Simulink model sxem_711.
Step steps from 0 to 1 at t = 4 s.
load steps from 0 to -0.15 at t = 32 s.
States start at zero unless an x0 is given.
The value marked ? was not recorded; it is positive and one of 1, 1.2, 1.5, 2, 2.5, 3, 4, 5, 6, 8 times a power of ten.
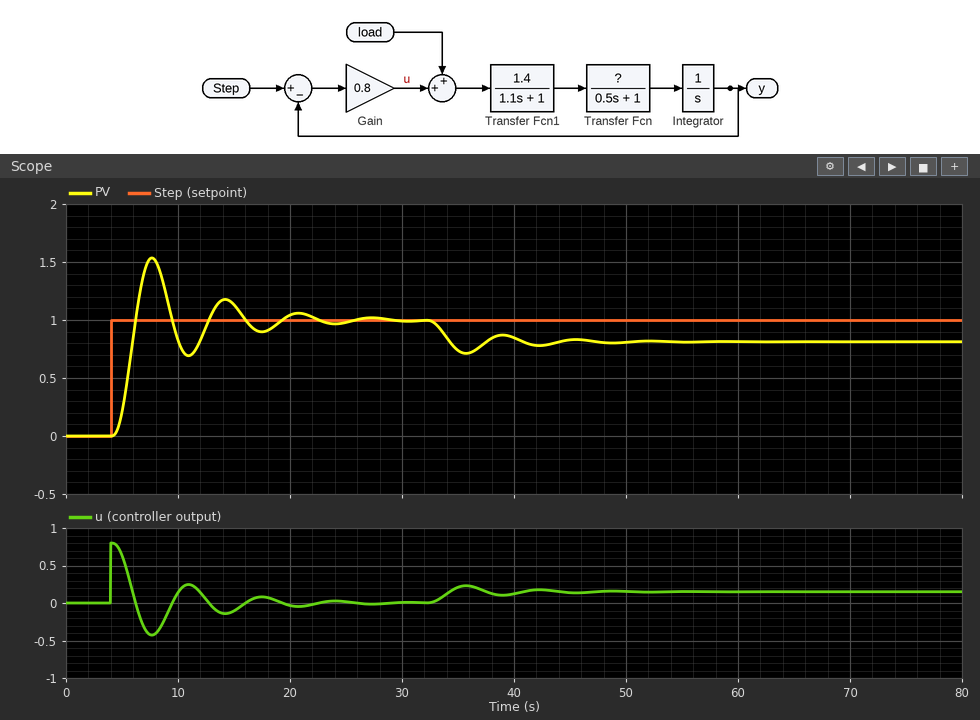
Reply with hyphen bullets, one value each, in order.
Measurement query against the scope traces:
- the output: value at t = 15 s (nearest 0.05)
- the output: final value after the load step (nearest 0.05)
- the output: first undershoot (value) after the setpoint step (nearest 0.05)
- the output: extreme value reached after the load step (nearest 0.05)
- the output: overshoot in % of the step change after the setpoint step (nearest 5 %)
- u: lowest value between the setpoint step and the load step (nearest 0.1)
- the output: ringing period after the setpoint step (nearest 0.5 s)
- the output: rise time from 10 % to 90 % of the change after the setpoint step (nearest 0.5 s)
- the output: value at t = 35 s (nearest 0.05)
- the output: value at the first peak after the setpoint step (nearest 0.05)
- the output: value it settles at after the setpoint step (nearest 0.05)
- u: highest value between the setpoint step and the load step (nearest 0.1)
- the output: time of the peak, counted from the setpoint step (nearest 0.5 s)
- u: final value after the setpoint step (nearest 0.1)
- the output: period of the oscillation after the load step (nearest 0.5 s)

- 1.15
- 0.80
- 0.70
- 0.70
- 55 %
- -0.4
- 6.5 s
- 1.5 s
- 0.75
- 1.55
- 1.00
- 0.8
- 3.5 s
- 0.0
- 6.5 s
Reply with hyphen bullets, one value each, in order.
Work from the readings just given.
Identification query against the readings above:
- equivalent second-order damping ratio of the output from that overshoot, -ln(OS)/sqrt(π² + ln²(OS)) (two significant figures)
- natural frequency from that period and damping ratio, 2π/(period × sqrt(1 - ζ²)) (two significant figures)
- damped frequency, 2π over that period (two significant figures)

- 0.19
- 0.98 rad/s
- 0.97 rad/s
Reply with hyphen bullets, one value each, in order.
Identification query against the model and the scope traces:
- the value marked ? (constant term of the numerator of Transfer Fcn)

- 1.2
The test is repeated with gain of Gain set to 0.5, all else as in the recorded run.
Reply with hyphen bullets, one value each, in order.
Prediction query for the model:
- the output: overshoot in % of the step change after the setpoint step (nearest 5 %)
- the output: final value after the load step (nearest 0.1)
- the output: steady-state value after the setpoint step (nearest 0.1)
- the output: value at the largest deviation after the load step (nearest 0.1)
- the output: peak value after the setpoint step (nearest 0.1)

- 35 %
- 0.7
- 1.0
- 0.6
- 1.3
